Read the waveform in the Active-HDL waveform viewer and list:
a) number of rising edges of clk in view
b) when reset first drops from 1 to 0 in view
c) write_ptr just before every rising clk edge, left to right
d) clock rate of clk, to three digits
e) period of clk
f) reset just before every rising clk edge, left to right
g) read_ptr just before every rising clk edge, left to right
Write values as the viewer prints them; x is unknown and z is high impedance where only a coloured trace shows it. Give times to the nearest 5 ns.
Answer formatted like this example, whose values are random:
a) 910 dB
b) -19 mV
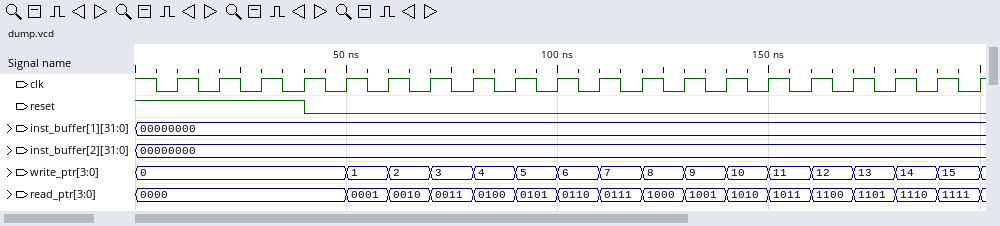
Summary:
a) 20
b) 40 ns
c) 0, 0, 0, 0, 0, 1, 2, 3, 4, 5, 6, 7, 8, 9, 10, 11, 12, 13, 14, 15
d) 100 MHz
e) 10 ns
f) 1 1 1 1 0 0 0 0 0 0 0 0 0 0 0 0 0 0 0 0
g) 0000, 0000, 0000, 0000, 0000, 0001, 0010, 0011, 0100, 0101, 0110, 0111, 1000, 1001, 1010, 1011, 1100, 1101, 1110, 1111
